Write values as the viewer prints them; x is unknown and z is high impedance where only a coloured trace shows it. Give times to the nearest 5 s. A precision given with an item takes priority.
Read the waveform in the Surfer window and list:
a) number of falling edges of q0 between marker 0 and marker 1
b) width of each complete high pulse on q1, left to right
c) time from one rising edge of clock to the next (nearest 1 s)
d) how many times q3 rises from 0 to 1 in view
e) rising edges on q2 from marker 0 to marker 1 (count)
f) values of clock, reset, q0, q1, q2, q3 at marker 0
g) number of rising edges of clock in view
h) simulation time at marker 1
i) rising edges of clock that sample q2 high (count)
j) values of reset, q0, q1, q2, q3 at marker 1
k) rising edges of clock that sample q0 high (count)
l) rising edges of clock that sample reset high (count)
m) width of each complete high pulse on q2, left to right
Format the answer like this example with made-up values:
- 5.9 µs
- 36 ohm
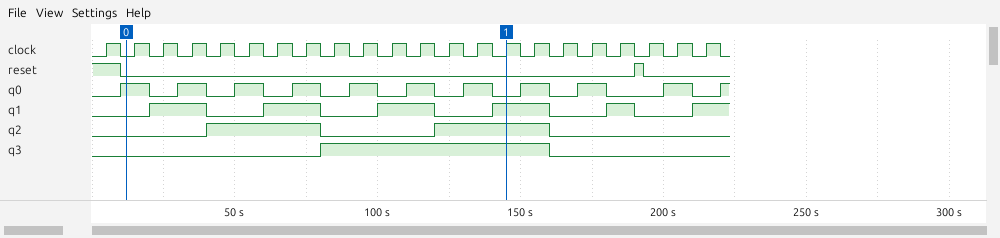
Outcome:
- 7
- 20 s, 20 s, 20 s, 20 s, 10 s
- 10 s
- 1
- 2
- clock=0, reset=0, q0=1, q1=0, q2=0, q3=0
- 22
- 145 s
- 8
- reset=0, q0=0, q1=1, q2=1, q3=1
- 10
- 1
- 40 s, 40 s
